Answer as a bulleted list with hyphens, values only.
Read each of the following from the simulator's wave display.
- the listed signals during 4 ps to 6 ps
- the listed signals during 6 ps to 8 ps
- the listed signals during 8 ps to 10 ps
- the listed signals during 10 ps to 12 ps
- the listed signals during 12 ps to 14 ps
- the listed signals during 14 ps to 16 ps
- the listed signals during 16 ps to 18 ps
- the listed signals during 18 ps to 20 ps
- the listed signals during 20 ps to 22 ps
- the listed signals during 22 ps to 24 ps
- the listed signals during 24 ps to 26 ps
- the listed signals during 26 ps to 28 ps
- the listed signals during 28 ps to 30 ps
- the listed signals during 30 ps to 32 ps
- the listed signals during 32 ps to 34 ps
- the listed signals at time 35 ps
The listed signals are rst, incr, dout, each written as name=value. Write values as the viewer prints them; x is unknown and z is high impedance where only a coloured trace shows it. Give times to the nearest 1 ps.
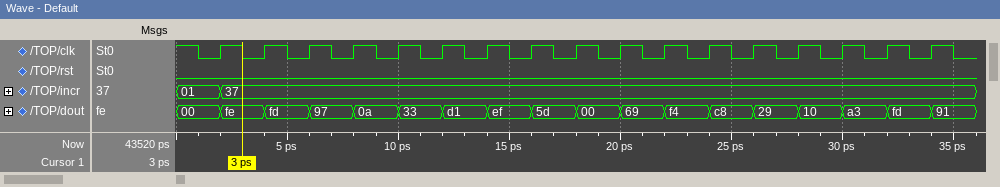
- rst=0, incr=37, dout=fd
- rst=0, incr=37, dout=97
- rst=0, incr=37, dout=0a
- rst=0, incr=37, dout=33
- rst=0, incr=37, dout=d1
- rst=0, incr=37, dout=ef
- rst=0, incr=37, dout=5d
- rst=0, incr=37, dout=00
- rst=0, incr=37, dout=69
- rst=0, incr=37, dout=f4
- rst=0, incr=37, dout=c8
- rst=0, incr=37, dout=29
- rst=0, incr=37, dout=10
- rst=0, incr=37, dout=a3
- rst=0, incr=37, dout=fd
- rst=0, incr=37, dout=91
